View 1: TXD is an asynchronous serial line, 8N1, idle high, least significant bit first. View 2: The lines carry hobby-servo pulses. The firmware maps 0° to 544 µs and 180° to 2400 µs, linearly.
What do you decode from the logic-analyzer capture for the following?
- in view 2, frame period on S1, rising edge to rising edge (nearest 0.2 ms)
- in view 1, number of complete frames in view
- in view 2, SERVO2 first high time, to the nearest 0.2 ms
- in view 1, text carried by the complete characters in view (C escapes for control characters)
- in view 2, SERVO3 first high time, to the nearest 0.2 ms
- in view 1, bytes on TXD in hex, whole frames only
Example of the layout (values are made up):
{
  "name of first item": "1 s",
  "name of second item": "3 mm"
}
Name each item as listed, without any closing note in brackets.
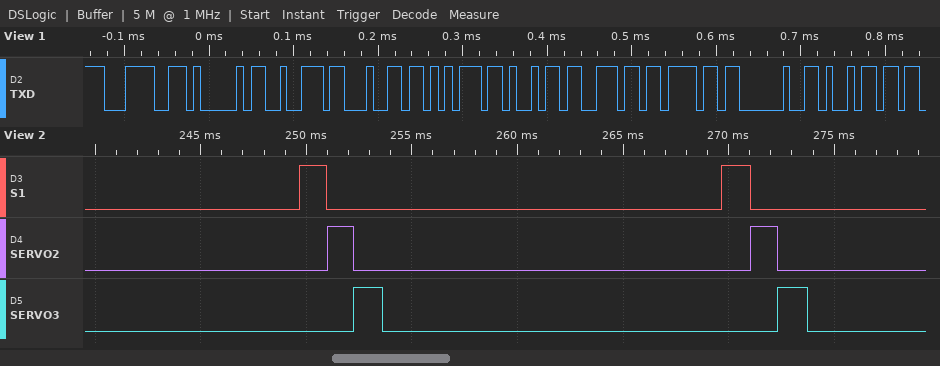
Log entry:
{
  "in view 2, frame period on S1, rising edge to rising edge": "20.0 ms",
  "in view 1, number of complete frames in view": "10",
  "in view 2, SERVO2 first high time, to the nearest 0.2 ms": "1.2 ms",
  "in view 1, text carried by the complete characters in view": "\"<Arduino i\"",
  "in view 2, SERVO3 first high time, to the nearest 0.2 ms": "1.4 ms",
  "in view 1, bytes on TXD in hex, whole frames only": "3C 41 72 64 75 69 6E 6F 20 69"
}
